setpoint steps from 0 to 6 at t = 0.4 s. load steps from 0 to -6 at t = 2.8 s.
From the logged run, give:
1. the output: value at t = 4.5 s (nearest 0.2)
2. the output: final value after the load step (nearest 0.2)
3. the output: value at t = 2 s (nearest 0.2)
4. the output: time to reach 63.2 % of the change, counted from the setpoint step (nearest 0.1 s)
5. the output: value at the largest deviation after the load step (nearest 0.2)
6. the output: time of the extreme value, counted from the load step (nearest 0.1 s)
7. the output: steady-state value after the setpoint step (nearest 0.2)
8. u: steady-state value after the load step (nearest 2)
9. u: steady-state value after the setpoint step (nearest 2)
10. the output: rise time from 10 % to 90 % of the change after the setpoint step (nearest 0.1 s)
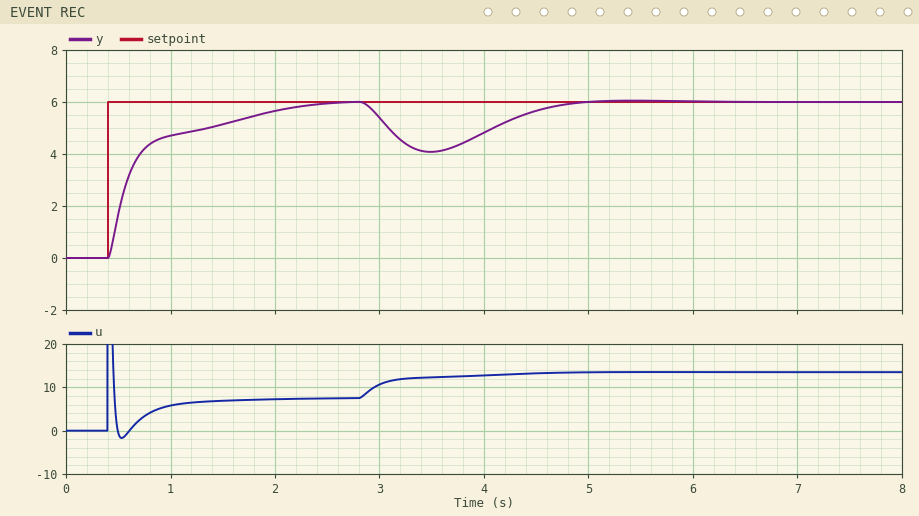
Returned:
5.6
6.0
5.6
0.3 s
4.0
0.7 s
6.0
14
8
1.3 s
